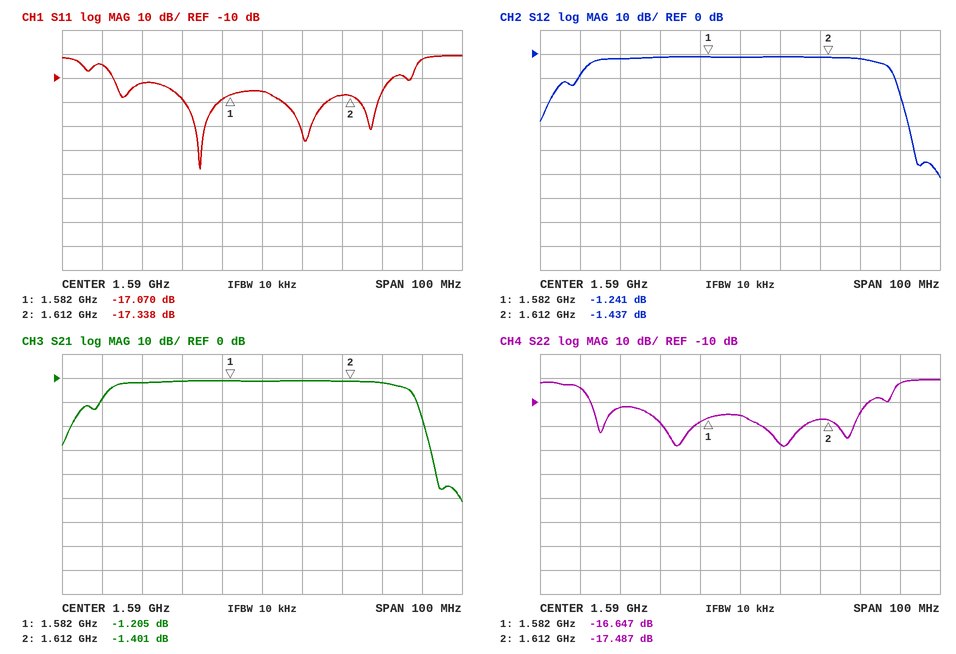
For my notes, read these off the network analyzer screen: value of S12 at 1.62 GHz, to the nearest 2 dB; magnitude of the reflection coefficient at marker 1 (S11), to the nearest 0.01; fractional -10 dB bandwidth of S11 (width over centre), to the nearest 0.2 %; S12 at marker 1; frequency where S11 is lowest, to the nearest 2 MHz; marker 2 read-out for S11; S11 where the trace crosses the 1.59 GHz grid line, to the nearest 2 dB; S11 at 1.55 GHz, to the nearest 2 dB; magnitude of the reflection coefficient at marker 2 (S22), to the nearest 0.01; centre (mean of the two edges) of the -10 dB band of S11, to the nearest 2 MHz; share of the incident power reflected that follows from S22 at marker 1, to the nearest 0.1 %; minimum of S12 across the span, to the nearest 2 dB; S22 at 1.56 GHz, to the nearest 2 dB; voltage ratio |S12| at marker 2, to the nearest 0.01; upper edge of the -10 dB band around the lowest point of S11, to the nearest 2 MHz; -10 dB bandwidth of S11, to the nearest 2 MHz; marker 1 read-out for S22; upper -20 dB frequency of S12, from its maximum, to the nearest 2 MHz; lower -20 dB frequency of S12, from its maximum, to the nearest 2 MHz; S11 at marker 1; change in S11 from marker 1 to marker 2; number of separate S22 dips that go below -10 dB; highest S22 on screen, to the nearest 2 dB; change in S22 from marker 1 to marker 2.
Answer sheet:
-2 dB
0.14
4.4 %
-1.241 dB
1.574 GHz
-17.338 dB
-16 dB
-4 dB
0.13
1.588 GHz
2.2 %
-52 dB
-12 dB
0.85
1.622 GHz
70 MHz
-16.647 dB
1.630 GHz
1.542 GHz
-17.070 dB
-0.268 dB
4
0 dB
-0.840 dB
